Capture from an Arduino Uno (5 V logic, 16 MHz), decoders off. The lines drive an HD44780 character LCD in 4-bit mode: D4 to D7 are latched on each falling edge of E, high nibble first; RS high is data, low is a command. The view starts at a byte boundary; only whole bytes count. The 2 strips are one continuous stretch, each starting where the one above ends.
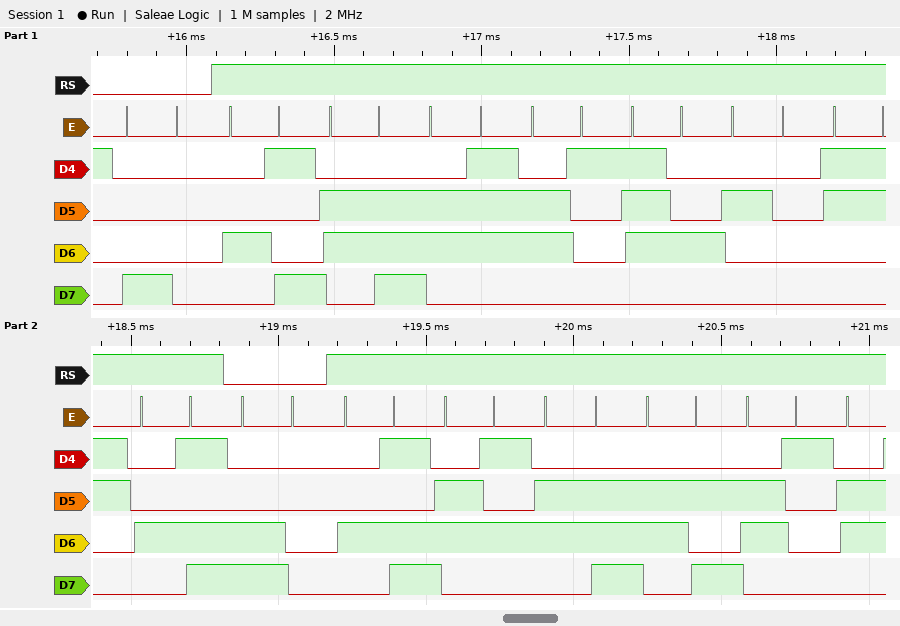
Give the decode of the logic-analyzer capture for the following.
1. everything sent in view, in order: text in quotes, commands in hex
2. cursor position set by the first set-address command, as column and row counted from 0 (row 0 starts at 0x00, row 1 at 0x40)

0x80 "Ingat 3M" 0xC0 "Menja"
column 0, row 0
